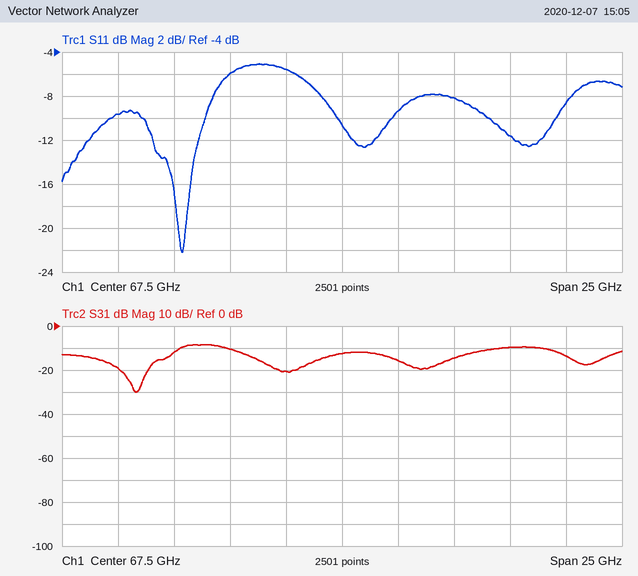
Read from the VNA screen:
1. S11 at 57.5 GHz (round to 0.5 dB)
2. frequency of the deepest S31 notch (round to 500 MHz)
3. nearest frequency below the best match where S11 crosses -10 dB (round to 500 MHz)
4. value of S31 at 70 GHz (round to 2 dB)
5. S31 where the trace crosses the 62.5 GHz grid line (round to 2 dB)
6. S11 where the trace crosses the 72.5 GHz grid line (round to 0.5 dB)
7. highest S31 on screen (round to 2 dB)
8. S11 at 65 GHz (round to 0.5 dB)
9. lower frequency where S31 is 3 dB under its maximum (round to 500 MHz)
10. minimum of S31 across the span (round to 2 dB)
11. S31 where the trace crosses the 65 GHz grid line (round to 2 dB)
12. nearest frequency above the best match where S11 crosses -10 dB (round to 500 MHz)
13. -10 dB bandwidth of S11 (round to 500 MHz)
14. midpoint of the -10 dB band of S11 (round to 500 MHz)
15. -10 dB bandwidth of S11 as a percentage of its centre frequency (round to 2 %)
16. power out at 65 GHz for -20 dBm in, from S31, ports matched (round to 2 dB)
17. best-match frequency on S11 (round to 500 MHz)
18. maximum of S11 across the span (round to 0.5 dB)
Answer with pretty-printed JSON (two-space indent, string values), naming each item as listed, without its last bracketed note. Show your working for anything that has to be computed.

{
  "S11 at 57.5 GHz": "-9.5 dB",
  "frequency of the deepest S31 notch": "58.5 GHz",
  "nearest frequency below the best match where S11 crosses -10 dB": "58.5 GHz",
  "value of S31 at 70 GHz": "-16 dB",
  "S31 where the trace crosses the 62.5 GHz grid line": "-10 dB",
  "S11 where the trace crosses the 72.5 GHz grid line": "-8.0 dB",
  "highest S31 on screen": "-8 dB",
  "S11 at 65 GHz": "-5.5 dB",
  "lower frequency where S31 is 3 dB under its maximum": "60.0 GHz",
  "minimum of S31 across the span": "-30 dB",
  "S31 where the trace crosses the 65 GHz grid line": "-20 dB",
  "nearest frequency above the best match where S11 crosses -10 dB": "61.5 GHz",
  "-10 dB bandwidth of S11": "61.5 GHz − 58.5 GHz = 3.0 GHz",
  "midpoint of the -10 dB band of S11": "60.0 GHz",
  "-10 dB bandwidth of S11 as a percentage of its centre frequency": "3 GHz / 60 GHz ≈ 5.00 %, so 4 % to the nearest 2 %",
  "power out at 65 GHz for -20 dBm in, from S31, ports matched": "-20 dBm + (-20 dB) = -40 dBm",
  "best-match frequency on S11": "60.5 GHz",
  "maximum of S11 across the span": "-5.0 dB"
}
